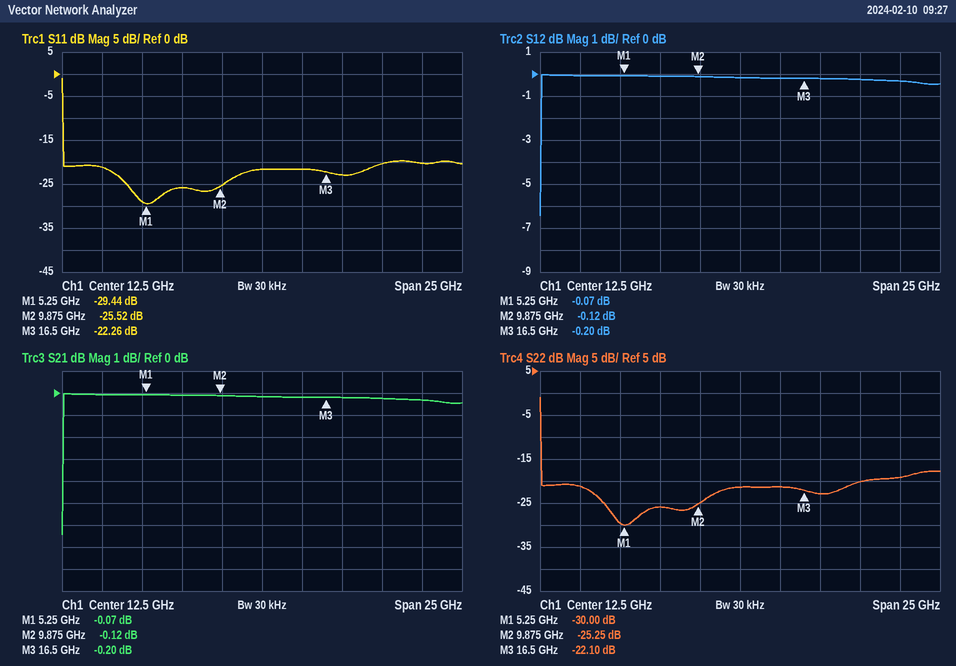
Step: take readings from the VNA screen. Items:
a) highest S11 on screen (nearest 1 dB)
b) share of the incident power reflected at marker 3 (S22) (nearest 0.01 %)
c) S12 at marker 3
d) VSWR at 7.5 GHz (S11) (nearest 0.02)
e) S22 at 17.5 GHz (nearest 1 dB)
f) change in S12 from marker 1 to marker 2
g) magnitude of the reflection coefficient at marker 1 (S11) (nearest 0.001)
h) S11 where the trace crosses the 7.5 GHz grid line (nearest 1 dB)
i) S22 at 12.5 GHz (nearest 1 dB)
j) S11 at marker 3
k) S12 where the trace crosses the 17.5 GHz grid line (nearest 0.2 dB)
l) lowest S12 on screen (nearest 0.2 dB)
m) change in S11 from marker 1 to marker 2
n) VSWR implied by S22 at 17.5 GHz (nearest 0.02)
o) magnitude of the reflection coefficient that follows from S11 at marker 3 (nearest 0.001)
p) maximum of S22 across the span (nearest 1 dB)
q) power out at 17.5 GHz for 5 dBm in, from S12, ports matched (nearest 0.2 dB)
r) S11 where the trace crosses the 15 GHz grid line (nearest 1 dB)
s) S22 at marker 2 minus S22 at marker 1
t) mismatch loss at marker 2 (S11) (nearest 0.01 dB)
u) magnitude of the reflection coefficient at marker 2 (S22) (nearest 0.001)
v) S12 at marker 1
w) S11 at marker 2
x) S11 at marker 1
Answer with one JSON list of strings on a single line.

["-1 dB", "0.62 %", "-0.20 dB", "1.10", "-23 dB", "-0.05 dB", "0.034", "-26 dB", "-21 dB", "-22.26 dB", "-0.2 dB", "-6.4 dB", "3.92 dB", "1.16", "0.077", "-1 dB", "4.8 dBm", "-22 dB", "4.75 dB", "0.01 dB", "0.055", "-0.07 dB", "-25.52 dB", "-29.44 dB"]
